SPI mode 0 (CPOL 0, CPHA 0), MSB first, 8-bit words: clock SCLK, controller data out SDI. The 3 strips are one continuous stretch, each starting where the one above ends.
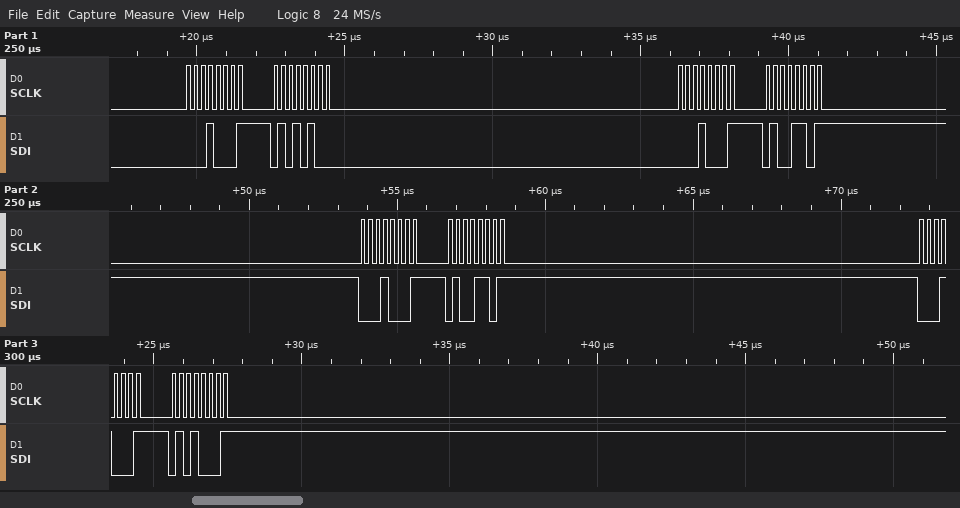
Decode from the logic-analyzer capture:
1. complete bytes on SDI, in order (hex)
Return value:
11 54 11 4D 11 4D 11 51
